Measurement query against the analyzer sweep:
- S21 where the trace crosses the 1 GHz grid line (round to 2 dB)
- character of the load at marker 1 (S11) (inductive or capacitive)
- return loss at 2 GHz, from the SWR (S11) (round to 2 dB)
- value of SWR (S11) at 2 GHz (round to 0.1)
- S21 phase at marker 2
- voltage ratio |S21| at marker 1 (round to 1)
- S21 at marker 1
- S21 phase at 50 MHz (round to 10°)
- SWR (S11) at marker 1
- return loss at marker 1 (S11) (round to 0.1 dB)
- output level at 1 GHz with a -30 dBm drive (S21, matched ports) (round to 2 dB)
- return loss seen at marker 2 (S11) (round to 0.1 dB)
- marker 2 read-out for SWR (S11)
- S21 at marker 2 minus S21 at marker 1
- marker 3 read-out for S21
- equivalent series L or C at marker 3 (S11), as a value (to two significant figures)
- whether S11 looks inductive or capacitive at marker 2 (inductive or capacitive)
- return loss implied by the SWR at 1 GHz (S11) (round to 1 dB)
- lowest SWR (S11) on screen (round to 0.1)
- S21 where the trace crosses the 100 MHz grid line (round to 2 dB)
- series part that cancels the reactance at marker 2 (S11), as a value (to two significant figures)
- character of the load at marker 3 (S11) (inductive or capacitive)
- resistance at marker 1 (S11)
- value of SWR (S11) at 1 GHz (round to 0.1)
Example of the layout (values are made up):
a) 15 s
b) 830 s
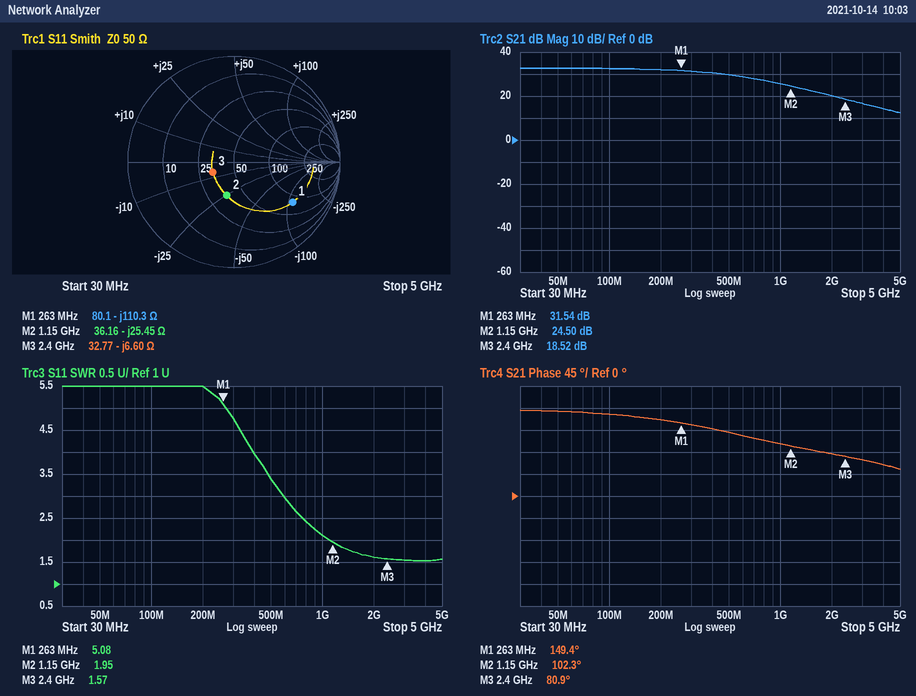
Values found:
a) 26 dB
b) capacitive
c) 12 dB
d) 1.6
e) 102.3°
f) 38
g) 31.54 dB
h) 170°
i) 5.08
j) 3.5 dB
k) -4 dBm
l) 9.8 dB
m) 1.95
n) -7.04 dB
o) 18.52 dB
p) 10 pF
q) capacitive
r) 9 dB
s) 1.5
t) 32 dB
u) 3.5 nH
v) capacitive
w) 80.1 Ω
x) 2.1
